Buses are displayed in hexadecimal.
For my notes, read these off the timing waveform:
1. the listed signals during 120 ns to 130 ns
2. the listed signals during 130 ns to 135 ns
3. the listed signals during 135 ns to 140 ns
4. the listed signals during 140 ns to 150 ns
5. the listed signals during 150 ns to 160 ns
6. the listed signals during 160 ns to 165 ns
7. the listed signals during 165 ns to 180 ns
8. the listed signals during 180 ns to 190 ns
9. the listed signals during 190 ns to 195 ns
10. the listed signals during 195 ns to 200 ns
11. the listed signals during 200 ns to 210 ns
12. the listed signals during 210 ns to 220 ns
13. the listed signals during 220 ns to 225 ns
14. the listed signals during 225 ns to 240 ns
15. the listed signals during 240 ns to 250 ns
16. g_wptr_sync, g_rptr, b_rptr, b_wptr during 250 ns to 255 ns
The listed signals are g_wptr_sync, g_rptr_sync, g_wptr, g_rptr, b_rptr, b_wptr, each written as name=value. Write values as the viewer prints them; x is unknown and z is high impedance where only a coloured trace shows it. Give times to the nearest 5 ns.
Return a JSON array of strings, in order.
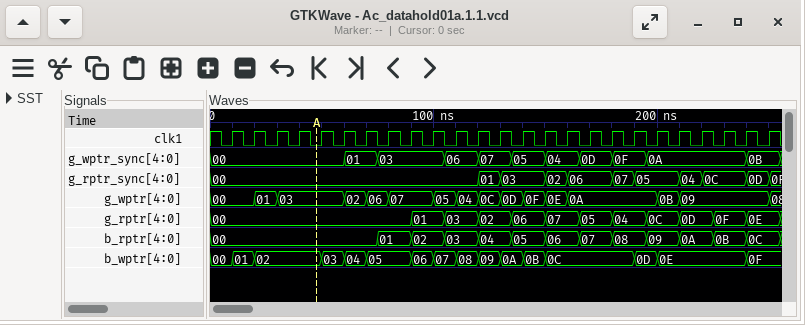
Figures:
["g_wptr_sync=07, g_rptr_sync=01, g_wptr=0C, g_rptr=02, b_rptr=04, b_wptr=09", "g_wptr_sync=07, g_rptr_sync=03, g_wptr=0D, g_rptr=02, b_rptr=04, b_wptr=0A", "g_wptr_sync=05, g_rptr_sync=03, g_wptr=0D, g_rptr=06, b_rptr=05, b_wptr=0A", "g_wptr_sync=05, g_rptr_sync=03, g_wptr=0F, g_rptr=06, b_rptr=05, b_wptr=0B", "g_wptr_sync=04, g_rptr_sync=02, g_wptr=0E, g_rptr=07, b_rptr=06, b_wptr=0C", "g_wptr_sync=04, g_rptr_sync=06, g_wptr=0A, g_rptr=07, b_rptr=06, b_wptr=0C", "g_wptr_sync=0D, g_rptr_sync=06, g_wptr=0A, g_rptr=05, b_rptr=07, b_wptr=0C", "g_wptr_sync=0F, g_rptr_sync=07, g_wptr=0A, g_rptr=04, b_rptr=08, b_wptr=0C", "g_wptr_sync=0F, g_rptr_sync=05, g_wptr=0A, g_rptr=04, b_rptr=08, b_wptr=0D", "g_wptr_sync=0A, g_rptr_sync=05, g_wptr=0A, g_rptr=0C, b_rptr=09, b_wptr=0D", "g_wptr_sync=0A, g_rptr_sync=05, g_wptr=0B, g_rptr=0C, b_rptr=09, b_wptr=0E", "g_wptr_sync=0A, g_rptr_sync=04, g_wptr=09, g_rptr=0D, b_rptr=0A, b_wptr=0E", "g_wptr_sync=0A, g_rptr_sync=0C, g_wptr=09, g_rptr=0D, b_rptr=0A, b_wptr=0E", "g_wptr_sync=0A, g_rptr_sync=0C, g_wptr=09, g_rptr=0F, b_rptr=0B, b_wptr=0E", "g_wptr_sync=0B, g_rptr_sync=0D, g_wptr=09, g_rptr=0E, b_rptr=0C, b_wptr=0F", "g_wptr_sync=0B, g_rptr=0E, b_rptr=0C, b_wptr=0F"]
